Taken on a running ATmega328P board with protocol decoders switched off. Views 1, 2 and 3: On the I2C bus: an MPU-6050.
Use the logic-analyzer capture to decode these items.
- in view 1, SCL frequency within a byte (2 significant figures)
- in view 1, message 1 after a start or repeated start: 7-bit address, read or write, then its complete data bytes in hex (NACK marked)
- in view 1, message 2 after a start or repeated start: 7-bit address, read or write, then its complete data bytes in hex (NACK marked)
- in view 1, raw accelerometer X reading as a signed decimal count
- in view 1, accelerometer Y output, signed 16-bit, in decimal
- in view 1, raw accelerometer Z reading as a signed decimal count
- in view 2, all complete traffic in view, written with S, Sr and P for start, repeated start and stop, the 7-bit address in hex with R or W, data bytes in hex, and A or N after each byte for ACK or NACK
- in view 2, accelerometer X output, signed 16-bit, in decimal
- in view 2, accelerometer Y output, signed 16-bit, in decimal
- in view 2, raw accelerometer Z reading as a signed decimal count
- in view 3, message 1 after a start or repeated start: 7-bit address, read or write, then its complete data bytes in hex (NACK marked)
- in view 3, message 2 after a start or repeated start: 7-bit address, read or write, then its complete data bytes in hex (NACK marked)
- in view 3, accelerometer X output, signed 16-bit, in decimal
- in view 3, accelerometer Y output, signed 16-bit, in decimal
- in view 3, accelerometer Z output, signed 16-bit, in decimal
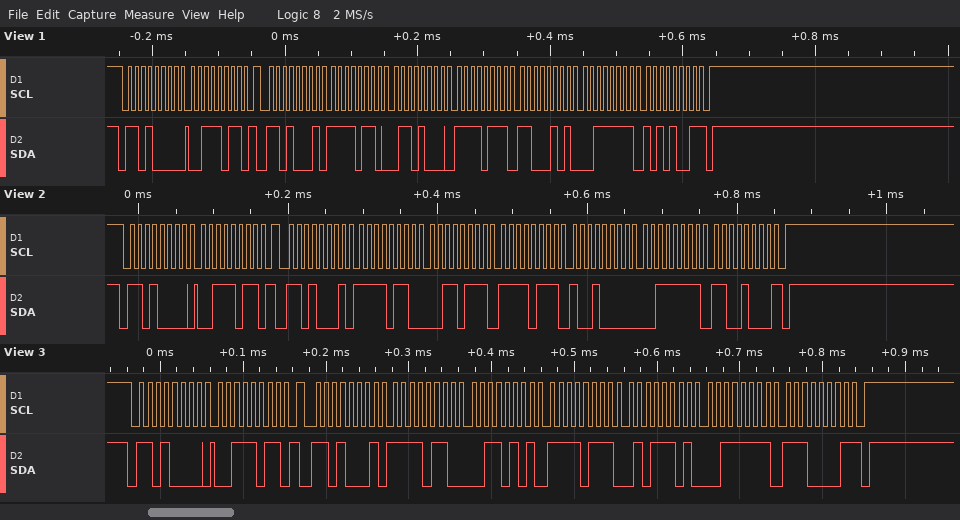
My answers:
100 kHz
0x68 write: 3B
0x68 read: F6 68 F7 C5 3F A9 NACK
-2456
-2107
16297
S 68W A 3B A Sr 68R A F6 A 37 A F7 A 90 A 3F A C8 N P
-2505
-2160
16328
0x68 write: 3B
0x68 read: F6 35 F7 5D 3F E1 NACK
-2507
-2211
16353
